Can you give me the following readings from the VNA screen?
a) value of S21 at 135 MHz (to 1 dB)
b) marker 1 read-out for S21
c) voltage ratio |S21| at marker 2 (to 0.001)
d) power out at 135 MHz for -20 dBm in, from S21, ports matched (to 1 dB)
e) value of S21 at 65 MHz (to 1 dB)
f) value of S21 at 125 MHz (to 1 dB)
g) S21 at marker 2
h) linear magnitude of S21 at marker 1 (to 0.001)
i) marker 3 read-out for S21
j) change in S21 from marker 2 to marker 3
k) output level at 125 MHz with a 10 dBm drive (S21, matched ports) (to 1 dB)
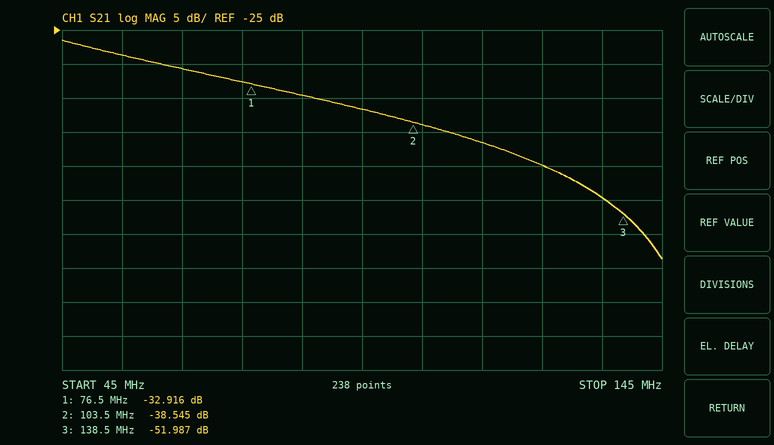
-50 dB
-32.916 dB
0.012
-70 dBm
-31 dB
-45 dB
-38.545 dB
0.023
-51.987 dB
-13.442 dB
-35 dBm
